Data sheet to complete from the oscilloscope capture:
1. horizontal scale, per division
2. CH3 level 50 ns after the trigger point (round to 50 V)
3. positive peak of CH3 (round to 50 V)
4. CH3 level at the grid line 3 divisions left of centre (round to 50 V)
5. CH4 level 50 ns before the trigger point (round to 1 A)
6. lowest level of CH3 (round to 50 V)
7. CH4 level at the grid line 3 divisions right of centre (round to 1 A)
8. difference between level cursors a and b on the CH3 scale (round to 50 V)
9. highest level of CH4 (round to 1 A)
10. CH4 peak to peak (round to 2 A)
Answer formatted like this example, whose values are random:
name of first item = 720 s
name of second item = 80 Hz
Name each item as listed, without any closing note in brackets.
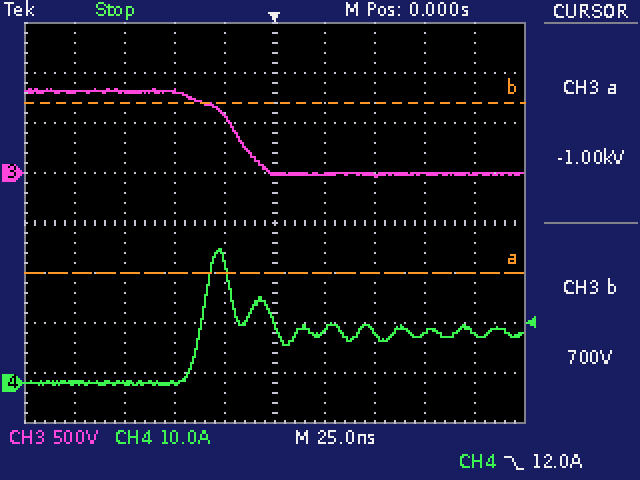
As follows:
horizontal scale, per division = 25 ns
CH3 level 50 ns after the trigger point = 0 V
positive peak of CH3 = 850 V
CH3 level at the grid line 3 divisions left of centre = 800 V
CH4 level 50 ns before the trigger point = 0 A
lowest level of CH3 = -50 V
CH4 level at the grid line 3 divisions right of centre = 10 A
difference between level cursors a and b on the CH3 scale = 1.70 kV
highest level of CH4 = 27 A
CH4 peak to peak = 28 A
